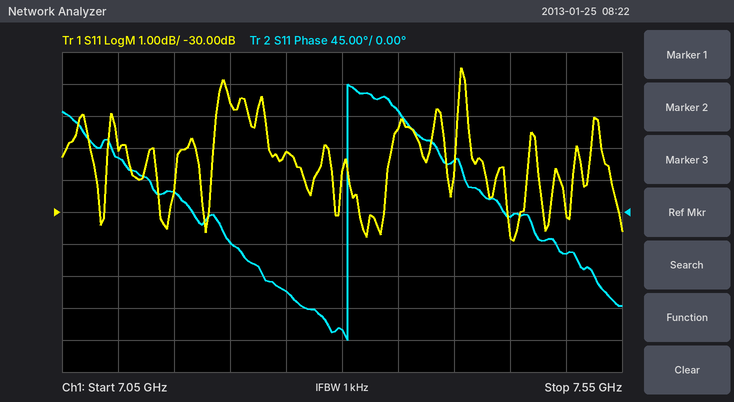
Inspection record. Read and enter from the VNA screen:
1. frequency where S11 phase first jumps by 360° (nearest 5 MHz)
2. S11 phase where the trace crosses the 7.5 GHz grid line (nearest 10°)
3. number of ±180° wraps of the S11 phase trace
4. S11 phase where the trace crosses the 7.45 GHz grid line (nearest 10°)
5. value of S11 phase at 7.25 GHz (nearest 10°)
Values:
7.305 GHz
-60°
1
-10°
-110°
